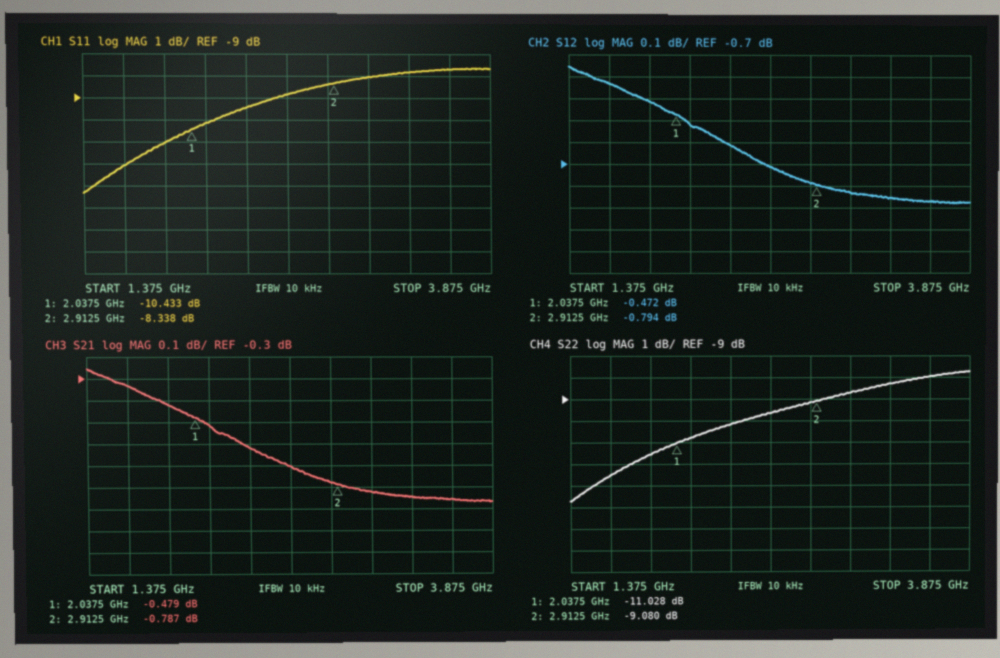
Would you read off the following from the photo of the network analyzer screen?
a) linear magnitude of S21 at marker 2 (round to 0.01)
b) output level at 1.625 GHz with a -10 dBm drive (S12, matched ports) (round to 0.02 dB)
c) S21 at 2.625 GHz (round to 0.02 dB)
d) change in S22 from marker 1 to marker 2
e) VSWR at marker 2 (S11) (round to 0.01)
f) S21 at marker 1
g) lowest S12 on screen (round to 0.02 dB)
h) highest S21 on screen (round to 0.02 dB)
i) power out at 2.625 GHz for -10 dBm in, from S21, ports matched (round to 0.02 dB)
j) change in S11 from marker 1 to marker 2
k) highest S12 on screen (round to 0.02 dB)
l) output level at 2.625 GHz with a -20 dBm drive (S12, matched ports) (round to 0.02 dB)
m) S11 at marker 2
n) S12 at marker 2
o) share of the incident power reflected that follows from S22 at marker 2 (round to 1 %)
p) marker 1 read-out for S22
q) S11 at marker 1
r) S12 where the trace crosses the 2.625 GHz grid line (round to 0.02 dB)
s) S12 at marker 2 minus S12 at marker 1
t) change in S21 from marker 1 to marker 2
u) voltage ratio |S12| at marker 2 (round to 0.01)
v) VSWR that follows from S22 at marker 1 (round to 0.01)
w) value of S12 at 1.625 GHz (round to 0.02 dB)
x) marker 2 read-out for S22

0.91
-10.34 dBm
-0.70 dB
1.948 dB
2.24
-0.479 dB
-0.88 dB
-0.26 dB
-10.70 dBm
2.095 dB
-0.26 dB
-20.72 dBm
-8.338 dB
-0.794 dB
12 %
-11.028 dB
-10.433 dB
-0.72 dB
-0.322 dB
-0.308 dB
0.91
1.78
-0.34 dB
-9.080 dB
